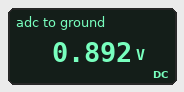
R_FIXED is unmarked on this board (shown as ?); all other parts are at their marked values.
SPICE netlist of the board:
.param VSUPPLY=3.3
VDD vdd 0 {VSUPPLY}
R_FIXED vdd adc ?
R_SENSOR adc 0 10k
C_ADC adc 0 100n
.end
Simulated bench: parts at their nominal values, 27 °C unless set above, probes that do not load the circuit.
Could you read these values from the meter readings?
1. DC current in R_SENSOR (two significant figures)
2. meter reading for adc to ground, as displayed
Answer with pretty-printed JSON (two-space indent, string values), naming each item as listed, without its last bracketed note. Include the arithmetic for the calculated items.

{
  "DC current in R_SENSOR": "(892 mV) / 10 kΩ = 89 µA",
  "meter reading for adc to ground, as displayed": "0.892 V"
}
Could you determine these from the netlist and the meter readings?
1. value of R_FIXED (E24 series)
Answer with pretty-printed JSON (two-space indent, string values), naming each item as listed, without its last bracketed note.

{
  "value of R_FIXED": "27 kΩ"
}
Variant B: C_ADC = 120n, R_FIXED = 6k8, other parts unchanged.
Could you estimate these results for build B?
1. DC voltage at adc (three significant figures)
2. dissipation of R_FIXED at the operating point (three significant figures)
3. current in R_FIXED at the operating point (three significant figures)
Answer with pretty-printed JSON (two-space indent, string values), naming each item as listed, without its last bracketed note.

{
  "DC voltage at adc": "1.96 V",
  "dissipation of R_FIXED at the operating point": "262 µW",
  "current in R_FIXED at the operating point": "196 µA"
}
